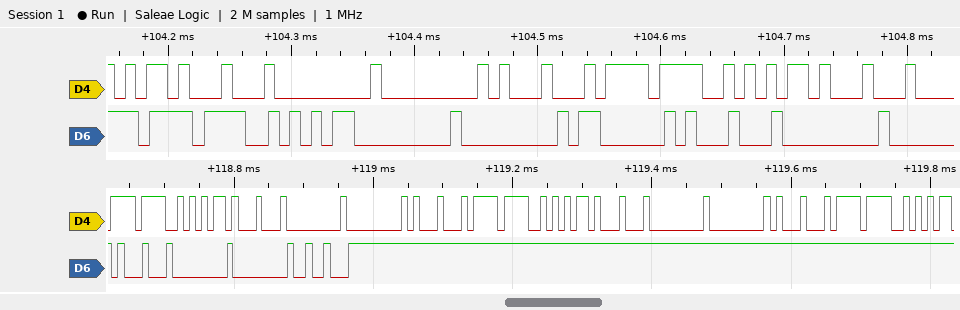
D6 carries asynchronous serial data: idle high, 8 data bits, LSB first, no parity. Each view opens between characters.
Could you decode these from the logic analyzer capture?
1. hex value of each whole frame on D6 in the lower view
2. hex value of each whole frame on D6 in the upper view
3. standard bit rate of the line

11, 00, 00, 12
EF, AA, 00, 00, 03, 11, 00
115200 baud
